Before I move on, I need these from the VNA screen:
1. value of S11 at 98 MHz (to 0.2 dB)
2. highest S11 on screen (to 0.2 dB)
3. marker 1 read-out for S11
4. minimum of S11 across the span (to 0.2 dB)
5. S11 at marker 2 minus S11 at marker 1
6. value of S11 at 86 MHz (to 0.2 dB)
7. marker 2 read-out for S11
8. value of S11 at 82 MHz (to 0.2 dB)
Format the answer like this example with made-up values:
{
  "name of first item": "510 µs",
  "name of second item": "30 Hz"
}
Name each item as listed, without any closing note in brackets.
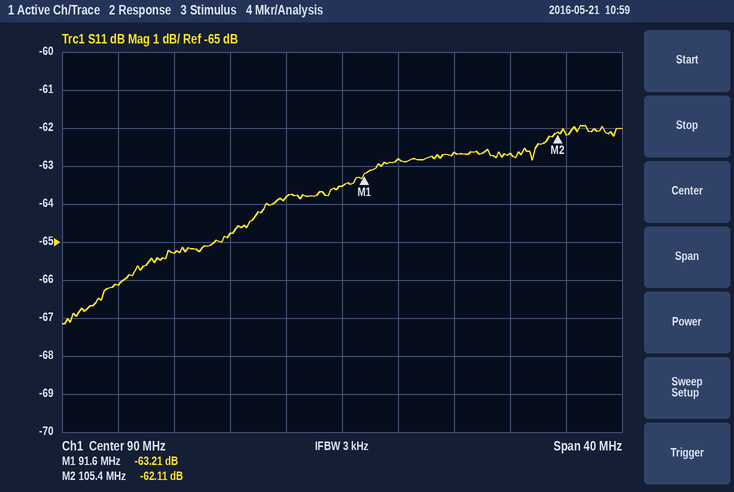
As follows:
{
  "value of S11 at 98 MHz": "-62.6 dB",
  "highest S11 on screen": "-62.0 dB",
  "marker 1 read-out for S11": "-63.21 dB",
  "minimum of S11 across the span": "-67.2 dB",
  "S11 at marker 2 minus S11 at marker 1": "1.10 dB",
  "value of S11 at 86 MHz": "-63.8 dB",
  "marker 2 read-out for S11": "-62.11 dB",
  "value of S11 at 82 MHz": "-64.8 dB"
}
